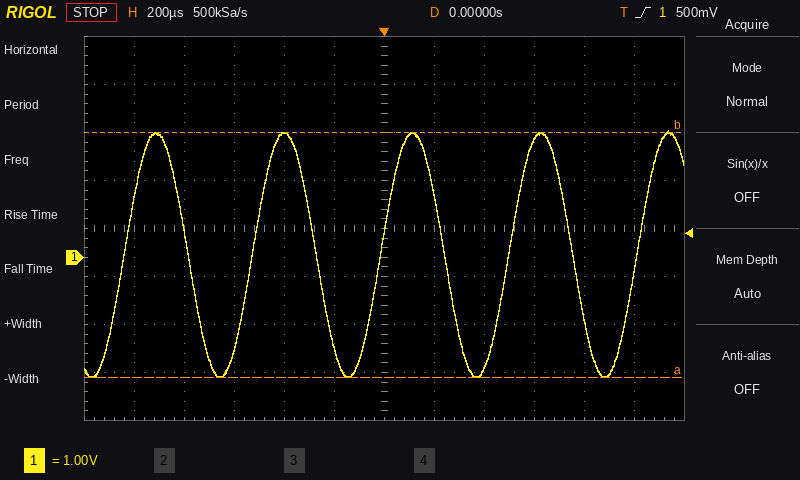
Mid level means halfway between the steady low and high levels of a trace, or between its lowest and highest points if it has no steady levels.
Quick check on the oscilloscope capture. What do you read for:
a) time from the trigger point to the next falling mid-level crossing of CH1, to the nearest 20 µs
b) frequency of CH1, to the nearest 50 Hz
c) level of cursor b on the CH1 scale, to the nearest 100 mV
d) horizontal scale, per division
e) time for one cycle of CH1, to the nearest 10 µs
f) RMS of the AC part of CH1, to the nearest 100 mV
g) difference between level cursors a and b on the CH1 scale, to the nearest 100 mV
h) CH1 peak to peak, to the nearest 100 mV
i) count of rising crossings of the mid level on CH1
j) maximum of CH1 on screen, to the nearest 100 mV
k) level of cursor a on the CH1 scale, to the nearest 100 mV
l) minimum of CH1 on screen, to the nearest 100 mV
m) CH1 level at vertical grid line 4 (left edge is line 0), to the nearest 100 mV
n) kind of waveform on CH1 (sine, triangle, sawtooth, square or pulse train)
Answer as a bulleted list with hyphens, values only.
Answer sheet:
- 240 µs
- 1.95 kHz
- 2.6 V
- 200 µs
- 510 µs
- 1.8 V
- 5.1 V
- 5.1 V
- 5
- 2.6 V
- -2.5 V
- -2.5 V
- 2.6 V
- sine
